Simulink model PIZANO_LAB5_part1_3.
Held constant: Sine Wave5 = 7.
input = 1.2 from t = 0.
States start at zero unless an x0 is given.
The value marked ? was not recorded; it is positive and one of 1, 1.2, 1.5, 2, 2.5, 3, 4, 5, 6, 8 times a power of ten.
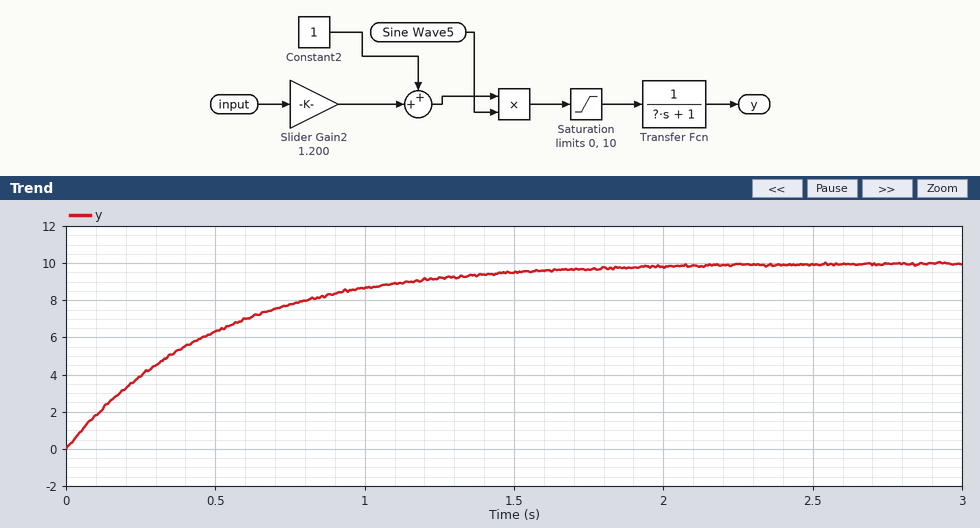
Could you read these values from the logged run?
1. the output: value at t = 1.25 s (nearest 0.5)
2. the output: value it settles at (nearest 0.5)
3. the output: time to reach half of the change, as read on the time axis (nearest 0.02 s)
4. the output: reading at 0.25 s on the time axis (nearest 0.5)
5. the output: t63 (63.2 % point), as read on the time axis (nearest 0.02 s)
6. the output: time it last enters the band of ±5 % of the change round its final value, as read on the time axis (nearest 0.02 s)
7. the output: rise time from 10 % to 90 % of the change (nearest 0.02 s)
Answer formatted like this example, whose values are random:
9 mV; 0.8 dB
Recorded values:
9.0; 10.0; 0.34 s; 4.0; 0.50 s; 1.50 s; 1.10 s
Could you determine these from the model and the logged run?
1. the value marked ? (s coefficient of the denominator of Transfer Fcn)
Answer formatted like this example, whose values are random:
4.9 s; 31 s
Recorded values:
0.5
